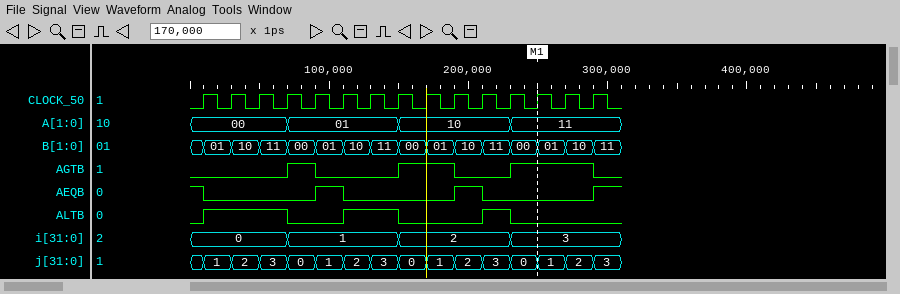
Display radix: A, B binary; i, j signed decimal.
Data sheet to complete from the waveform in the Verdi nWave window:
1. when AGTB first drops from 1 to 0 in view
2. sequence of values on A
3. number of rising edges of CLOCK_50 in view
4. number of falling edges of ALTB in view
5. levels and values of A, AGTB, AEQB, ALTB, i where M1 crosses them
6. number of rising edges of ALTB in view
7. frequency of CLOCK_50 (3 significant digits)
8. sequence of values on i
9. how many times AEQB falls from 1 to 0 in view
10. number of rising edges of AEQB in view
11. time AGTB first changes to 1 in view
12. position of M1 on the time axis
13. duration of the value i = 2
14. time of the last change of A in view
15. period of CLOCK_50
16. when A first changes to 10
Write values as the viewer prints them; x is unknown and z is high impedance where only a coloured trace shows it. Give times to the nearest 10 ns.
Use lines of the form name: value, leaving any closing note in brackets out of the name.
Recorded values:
when AGTB first drops from 1 to 0 in view: 90 ns
sequence of values on A: 00, 01, 10, 11
number of rising edges of CLOCK_50 in view: 15
number of falling edges of ALTB in view: 3
levels and values of A, AGTB, AEQB, ALTB, i where M1 crosses them: A=11, AGTB=1, AEQB=0, ALTB=0, i=3
number of rising edges of ALTB in view: 3
frequency of CLOCK_50: 50.0 MHz
sequence of values on i: 0, 1, 2, 3
how many times AEQB falls from 1 to 0 in view: 3
number of rising edges of AEQB in view: 3
time AGTB first changes to 1 in view: 70 ns
position of M1 on the time axis: 250 ns
duration of the value i = 2: 80 ns
time of the last change of A in view: 230 ns
period of CLOCK_50: 20 ns
when A first changes to 10: 150 ns
